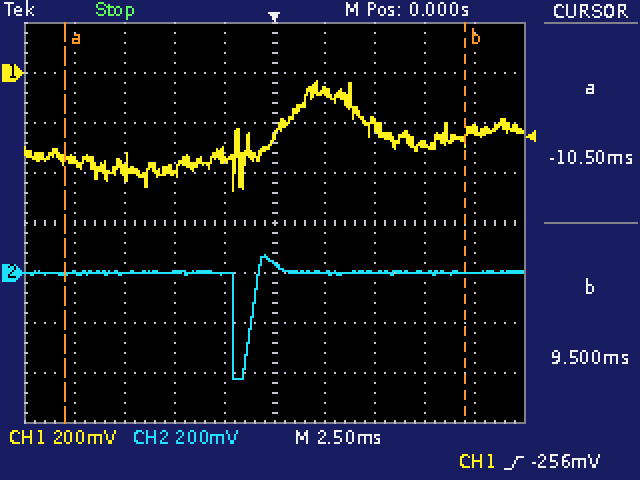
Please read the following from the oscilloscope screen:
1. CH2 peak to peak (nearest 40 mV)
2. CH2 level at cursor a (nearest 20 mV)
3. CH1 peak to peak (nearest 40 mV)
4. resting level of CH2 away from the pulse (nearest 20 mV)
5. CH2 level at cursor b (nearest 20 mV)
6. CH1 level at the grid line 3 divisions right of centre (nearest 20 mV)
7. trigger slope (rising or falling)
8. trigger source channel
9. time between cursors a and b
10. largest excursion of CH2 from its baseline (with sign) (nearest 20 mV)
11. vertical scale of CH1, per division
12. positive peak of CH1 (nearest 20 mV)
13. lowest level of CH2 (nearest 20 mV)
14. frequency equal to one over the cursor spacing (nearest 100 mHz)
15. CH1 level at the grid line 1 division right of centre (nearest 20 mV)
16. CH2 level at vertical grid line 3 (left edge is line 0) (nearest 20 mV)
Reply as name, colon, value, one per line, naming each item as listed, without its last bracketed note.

CH2 peak to peak: 480 mV
CH2 level at cursor a: 0 mV
CH1 peak to peak: 440 mV
resting level of CH2 away from the pulse: 0 mV
CH2 level at cursor b: 0 mV
CH1 level at the grid line 3 divisions right of centre: -280 mV
trigger slope: rising
trigger source channel: CH1
time between cursors a and b: 20.00 ms
largest excursion of CH2 from its baseline (with sign): -420 mV
vertical scale of CH1, per division: 200 mV
positive peak of CH1: -40 mV
lowest level of CH2: -420 mV
frequency equal to one over the cursor spacing: 50.0 Hz
CH1 level at the grid line 1 division right of centre: -80 mV
CH2 level at vertical grid line 3 (left edge is line 0): 0 mV
